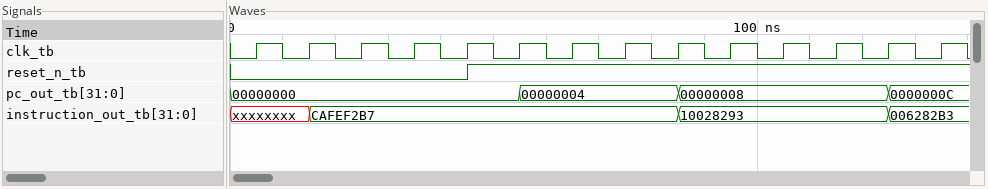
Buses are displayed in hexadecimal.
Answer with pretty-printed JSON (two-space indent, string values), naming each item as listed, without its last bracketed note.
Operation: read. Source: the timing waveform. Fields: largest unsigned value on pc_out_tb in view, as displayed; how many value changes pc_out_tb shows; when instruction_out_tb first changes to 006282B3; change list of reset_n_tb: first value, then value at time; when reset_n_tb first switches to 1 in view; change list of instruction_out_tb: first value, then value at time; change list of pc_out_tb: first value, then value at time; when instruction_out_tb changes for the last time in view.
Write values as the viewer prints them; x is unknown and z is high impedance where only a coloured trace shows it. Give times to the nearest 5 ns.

{
  "largest unsigned value on pc_out_tb in view, as displayed": "0000000C",
  "how many value changes pc_out_tb shows": "3",
  "when instruction_out_tb first changes to 006282B3": "125 ns",
  "change list of reset_n_tb: first value, then value at time": "0, 1 at 45 ns",
  "when reset_n_tb first switches to 1 in view": "45 ns",
  "change list of instruction_out_tb: first value, then value at time": "xxxxxxxx, CAFEF2B7 at 15 ns, 10028293 at 85 ns, 006282B3 at 125 ns",
  "change list of pc_out_tb: first value, then value at time": "00000000, 00000004 at 55 ns, 00000008 at 85 ns, 0000000C at 125 ns",
  "when instruction_out_tb changes for the last time in view": "125 ns"
}
